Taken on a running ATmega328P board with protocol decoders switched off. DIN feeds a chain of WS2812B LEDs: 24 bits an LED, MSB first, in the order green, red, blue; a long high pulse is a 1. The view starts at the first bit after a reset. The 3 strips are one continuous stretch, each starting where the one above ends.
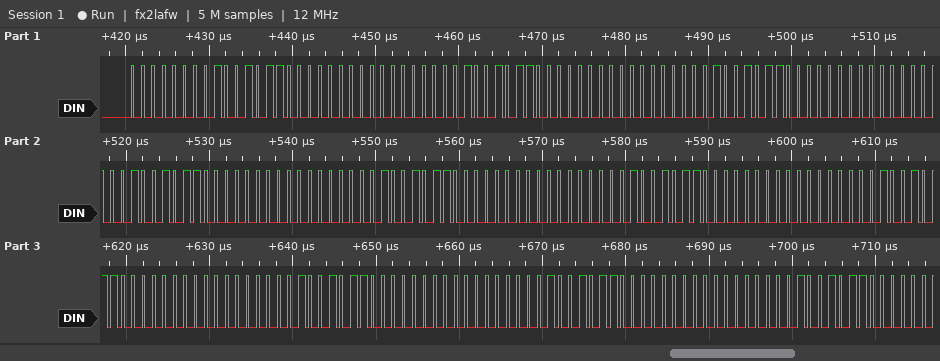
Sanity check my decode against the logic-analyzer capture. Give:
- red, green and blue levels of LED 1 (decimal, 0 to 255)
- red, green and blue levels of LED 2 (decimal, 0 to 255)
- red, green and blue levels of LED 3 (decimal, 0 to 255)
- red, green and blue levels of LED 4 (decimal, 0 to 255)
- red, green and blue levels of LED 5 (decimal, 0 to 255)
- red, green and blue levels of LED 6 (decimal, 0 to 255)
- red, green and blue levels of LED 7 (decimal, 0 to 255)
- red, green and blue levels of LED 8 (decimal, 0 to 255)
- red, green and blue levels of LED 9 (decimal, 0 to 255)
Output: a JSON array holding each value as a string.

["150, 0, 0", "150, 0, 0", "150, 0, 0", "150, 0, 0", "150, 0, 0", "150, 0, 0", "150, 0, 0", "150, 0, 0", "150, 0, 0"]
